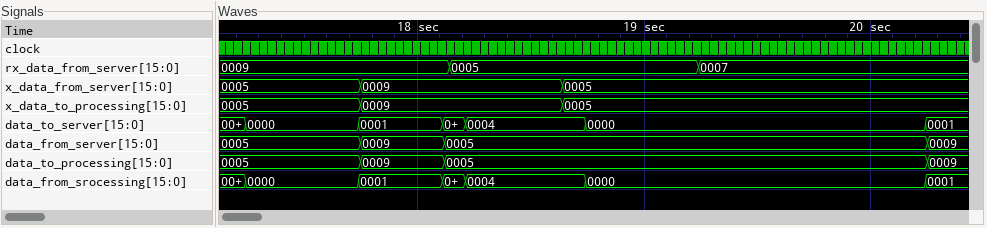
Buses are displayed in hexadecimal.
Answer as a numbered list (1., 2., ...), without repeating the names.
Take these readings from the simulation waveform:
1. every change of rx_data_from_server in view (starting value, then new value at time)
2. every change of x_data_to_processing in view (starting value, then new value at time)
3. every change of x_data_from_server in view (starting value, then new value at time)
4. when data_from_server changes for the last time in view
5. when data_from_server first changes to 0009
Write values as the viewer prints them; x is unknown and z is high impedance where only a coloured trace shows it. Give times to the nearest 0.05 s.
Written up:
1. 0009, 0005 at 18.15 s, 0007 at 19.25 s
2. 0005, 0009 at 17.75 s, 0005 at 18.65 s
3. 0005, 0009 at 17.75 s, 0005 at 18.65 s
4. 20.25 s
5. 17.75 s
